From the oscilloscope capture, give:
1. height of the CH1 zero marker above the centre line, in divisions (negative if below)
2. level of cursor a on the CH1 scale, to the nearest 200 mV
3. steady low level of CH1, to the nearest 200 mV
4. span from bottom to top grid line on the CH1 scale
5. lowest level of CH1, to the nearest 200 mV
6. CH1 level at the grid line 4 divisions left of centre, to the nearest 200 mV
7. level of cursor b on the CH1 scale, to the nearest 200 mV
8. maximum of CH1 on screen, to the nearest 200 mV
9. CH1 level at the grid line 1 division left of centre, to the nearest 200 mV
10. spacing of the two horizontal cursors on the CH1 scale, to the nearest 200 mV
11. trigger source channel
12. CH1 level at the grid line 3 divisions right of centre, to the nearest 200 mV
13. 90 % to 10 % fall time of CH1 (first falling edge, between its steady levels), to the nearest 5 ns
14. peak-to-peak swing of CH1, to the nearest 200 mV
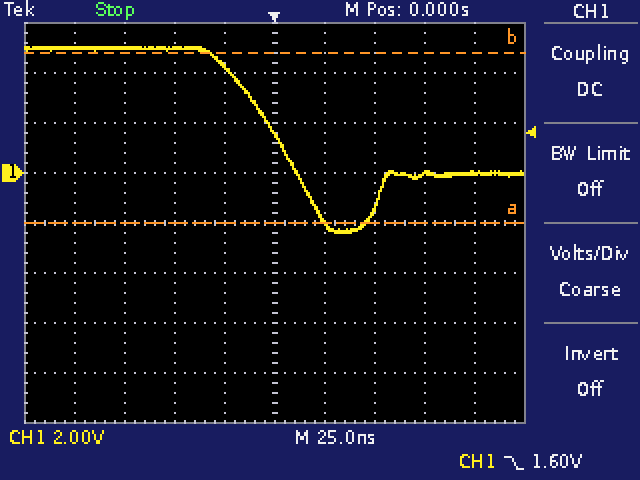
+1.0 div
-2.0 V
0.0 V
16 V
-2.4 V
5.0 V
4.8 V
5.0 V
4.2 V
6.8 V
CH1
0.0 V
35 ns
7.4 V
